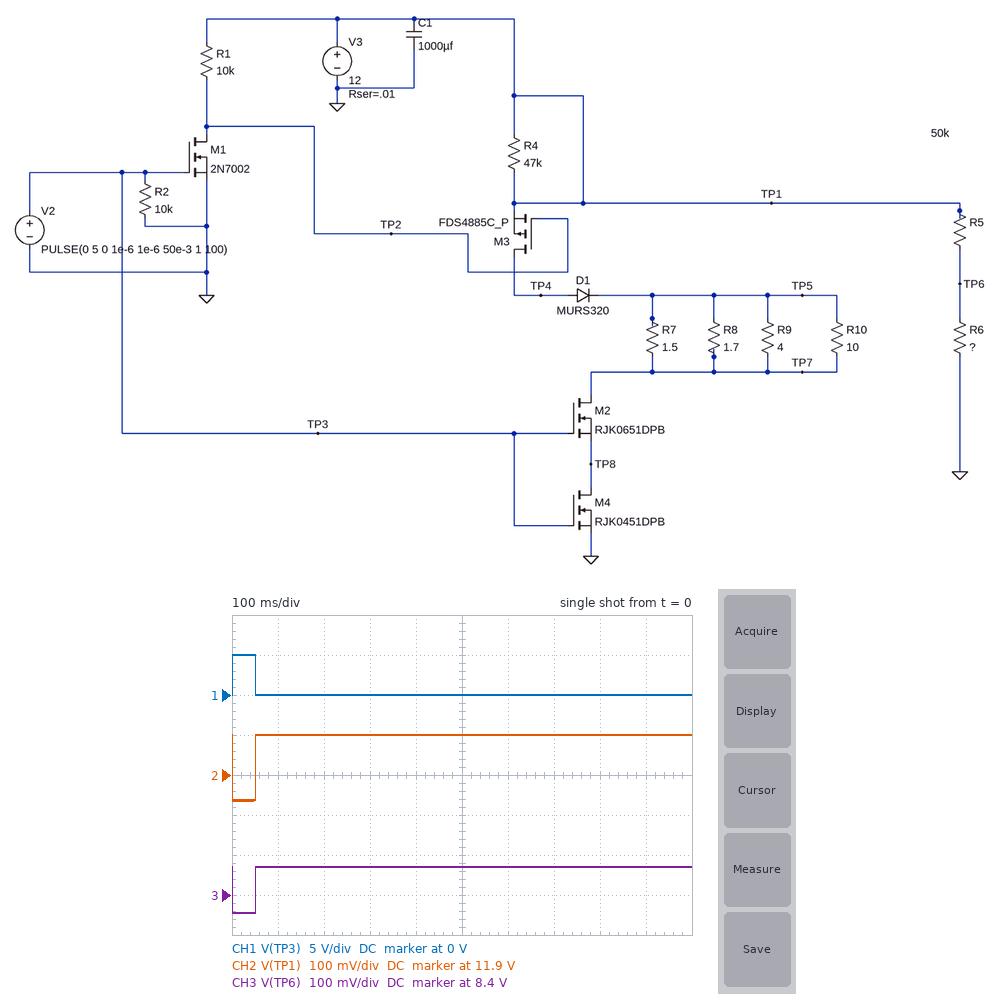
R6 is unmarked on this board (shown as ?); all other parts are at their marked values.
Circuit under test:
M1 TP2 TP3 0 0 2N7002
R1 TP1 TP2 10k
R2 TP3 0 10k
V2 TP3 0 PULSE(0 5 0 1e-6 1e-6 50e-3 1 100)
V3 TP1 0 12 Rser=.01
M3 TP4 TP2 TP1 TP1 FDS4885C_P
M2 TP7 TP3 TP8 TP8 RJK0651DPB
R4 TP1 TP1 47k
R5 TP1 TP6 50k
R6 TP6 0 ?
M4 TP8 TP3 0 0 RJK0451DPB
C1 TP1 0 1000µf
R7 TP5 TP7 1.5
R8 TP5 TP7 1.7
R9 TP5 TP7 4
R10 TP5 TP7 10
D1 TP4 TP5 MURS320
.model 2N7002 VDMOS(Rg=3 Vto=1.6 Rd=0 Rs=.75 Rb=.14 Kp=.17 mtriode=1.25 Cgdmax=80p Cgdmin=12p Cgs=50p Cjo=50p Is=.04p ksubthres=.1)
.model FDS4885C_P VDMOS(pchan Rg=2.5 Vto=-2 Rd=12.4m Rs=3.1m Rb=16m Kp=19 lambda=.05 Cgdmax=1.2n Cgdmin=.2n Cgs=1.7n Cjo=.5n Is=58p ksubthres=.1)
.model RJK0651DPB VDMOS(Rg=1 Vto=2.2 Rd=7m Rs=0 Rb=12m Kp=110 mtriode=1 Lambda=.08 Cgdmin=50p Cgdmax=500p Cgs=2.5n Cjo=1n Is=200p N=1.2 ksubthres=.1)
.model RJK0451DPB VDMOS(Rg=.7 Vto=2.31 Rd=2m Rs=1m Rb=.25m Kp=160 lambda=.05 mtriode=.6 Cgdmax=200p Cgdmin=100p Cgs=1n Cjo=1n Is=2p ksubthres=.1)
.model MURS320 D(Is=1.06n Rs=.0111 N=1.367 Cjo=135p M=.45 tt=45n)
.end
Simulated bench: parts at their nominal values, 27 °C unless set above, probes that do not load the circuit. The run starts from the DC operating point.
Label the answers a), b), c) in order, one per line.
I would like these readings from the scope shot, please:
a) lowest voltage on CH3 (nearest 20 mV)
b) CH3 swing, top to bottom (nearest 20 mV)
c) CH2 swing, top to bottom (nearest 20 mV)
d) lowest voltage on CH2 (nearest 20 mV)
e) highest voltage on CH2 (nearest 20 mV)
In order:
a) 8.36 V
b) 120 mV
c) 160 mV
d) 11.84 V
e) 12.00 V
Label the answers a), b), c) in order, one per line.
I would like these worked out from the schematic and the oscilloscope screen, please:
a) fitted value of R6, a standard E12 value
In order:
a) 120 kΩ
